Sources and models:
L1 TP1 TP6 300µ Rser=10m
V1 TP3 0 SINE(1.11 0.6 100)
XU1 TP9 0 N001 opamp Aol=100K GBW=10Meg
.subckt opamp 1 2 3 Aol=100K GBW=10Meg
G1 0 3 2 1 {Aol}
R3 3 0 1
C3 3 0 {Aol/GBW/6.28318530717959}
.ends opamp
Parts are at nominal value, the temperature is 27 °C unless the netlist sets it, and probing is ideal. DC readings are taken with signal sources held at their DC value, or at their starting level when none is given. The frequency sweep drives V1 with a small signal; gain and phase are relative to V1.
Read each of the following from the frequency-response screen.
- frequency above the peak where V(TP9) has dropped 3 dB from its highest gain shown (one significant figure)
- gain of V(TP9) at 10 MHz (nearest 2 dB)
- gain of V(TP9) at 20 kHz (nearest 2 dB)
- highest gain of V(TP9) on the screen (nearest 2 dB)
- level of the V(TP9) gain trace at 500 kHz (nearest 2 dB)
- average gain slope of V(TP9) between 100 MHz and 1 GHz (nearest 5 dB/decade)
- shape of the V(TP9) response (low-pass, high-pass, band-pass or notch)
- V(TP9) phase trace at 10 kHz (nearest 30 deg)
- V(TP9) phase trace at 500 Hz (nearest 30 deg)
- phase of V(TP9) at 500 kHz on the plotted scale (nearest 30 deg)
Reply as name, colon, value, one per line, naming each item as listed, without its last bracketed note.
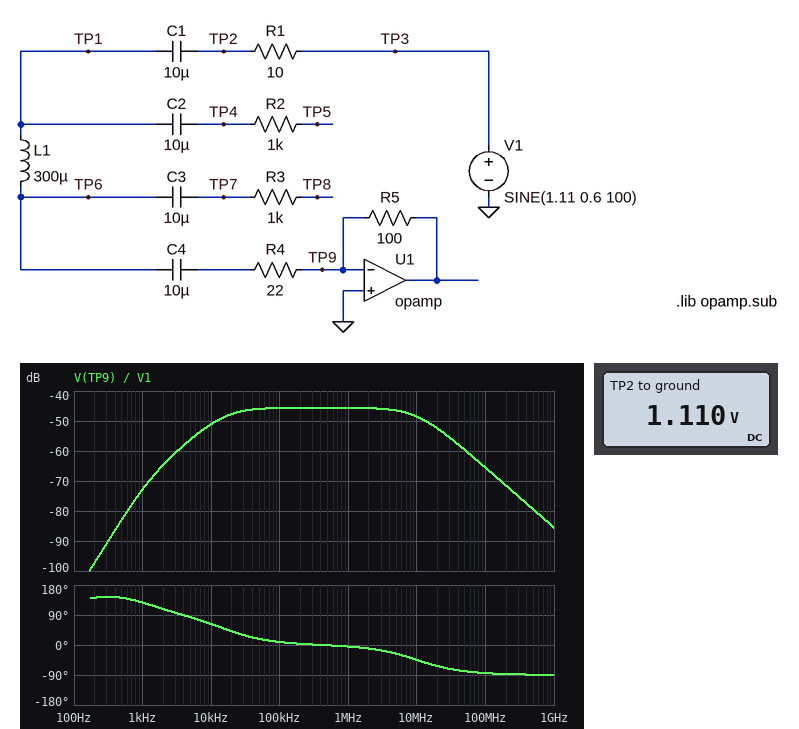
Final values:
frequency above the peak where V(TP9) has dropped 3 dB from its highest gain shown: 10 MHz
gain of V(TP9) at 10 MHz: -48 dB
gain of V(TP9) at 20 kHz: -48 dB
highest gain of V(TP9) on the screen: -46 dB
level of the V(TP9) gain trace at 500 kHz: -46 dB
average gain slope of V(TP9) between 100 MHz and 1 GHz: -20 dB/decade
shape of the V(TP9) response: band-pass
V(TP9) phase trace at 10 kHz: 60 deg
V(TP9) phase trace at 500 Hz: 150 deg
phase of V(TP9) at 500 kHz on the plotted scale: 0 deg
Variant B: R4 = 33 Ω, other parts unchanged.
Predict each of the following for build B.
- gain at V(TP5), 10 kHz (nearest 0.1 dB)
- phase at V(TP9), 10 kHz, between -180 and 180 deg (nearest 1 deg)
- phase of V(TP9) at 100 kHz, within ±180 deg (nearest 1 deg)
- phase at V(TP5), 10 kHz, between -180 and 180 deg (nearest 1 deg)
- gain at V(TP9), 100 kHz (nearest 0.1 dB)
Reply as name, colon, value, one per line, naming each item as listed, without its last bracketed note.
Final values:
gain at V(TP5), 10 kHz: -1.8 dB
phase at V(TP9), 10 kHz, between -180 and 180 deg: 69 deg
phase of V(TP9) at 100 kHz, within ±180 deg: 12 deg
phase at V(TP5), 10 kHz, between -180 and 180 deg: 8 deg
gain at V(TP9), 100 kHz: -45.8 dB
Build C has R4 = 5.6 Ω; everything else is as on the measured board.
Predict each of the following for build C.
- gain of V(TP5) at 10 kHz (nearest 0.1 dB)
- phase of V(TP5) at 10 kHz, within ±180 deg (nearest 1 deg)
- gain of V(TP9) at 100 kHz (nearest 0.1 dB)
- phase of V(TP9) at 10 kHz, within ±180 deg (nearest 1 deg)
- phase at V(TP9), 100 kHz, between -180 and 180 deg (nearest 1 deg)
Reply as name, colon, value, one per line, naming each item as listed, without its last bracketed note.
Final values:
gain of V(TP5) at 10 kHz: -1.7 dB
phase of V(TP5) at 10 kHz, within ±180 deg: 27 deg
gain of V(TP9) at 100 kHz: -45.6 dB
phase of V(TP9) at 10 kHz, within ±180 deg: 44 deg
phase at V(TP9), 100 kHz, between -180 and 180 deg: 4 deg
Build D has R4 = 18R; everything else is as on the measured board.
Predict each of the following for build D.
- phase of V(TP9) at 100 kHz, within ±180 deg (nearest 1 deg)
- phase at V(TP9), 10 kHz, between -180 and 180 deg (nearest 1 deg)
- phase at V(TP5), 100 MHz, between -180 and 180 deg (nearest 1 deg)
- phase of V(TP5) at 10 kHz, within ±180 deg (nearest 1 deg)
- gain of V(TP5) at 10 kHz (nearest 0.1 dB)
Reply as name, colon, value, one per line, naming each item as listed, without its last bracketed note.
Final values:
phase of V(TP9) at 100 kHz, within ±180 deg: 8 deg
phase at V(TP9), 10 kHz, between -180 and 180 deg: 60 deg
phase at V(TP5), 100 MHz, between -180 and 180 deg: 0 deg
phase of V(TP5) at 10 kHz, within ±180 deg: 15 deg
gain of V(TP5) at 10 kHz: -2.2 dB
